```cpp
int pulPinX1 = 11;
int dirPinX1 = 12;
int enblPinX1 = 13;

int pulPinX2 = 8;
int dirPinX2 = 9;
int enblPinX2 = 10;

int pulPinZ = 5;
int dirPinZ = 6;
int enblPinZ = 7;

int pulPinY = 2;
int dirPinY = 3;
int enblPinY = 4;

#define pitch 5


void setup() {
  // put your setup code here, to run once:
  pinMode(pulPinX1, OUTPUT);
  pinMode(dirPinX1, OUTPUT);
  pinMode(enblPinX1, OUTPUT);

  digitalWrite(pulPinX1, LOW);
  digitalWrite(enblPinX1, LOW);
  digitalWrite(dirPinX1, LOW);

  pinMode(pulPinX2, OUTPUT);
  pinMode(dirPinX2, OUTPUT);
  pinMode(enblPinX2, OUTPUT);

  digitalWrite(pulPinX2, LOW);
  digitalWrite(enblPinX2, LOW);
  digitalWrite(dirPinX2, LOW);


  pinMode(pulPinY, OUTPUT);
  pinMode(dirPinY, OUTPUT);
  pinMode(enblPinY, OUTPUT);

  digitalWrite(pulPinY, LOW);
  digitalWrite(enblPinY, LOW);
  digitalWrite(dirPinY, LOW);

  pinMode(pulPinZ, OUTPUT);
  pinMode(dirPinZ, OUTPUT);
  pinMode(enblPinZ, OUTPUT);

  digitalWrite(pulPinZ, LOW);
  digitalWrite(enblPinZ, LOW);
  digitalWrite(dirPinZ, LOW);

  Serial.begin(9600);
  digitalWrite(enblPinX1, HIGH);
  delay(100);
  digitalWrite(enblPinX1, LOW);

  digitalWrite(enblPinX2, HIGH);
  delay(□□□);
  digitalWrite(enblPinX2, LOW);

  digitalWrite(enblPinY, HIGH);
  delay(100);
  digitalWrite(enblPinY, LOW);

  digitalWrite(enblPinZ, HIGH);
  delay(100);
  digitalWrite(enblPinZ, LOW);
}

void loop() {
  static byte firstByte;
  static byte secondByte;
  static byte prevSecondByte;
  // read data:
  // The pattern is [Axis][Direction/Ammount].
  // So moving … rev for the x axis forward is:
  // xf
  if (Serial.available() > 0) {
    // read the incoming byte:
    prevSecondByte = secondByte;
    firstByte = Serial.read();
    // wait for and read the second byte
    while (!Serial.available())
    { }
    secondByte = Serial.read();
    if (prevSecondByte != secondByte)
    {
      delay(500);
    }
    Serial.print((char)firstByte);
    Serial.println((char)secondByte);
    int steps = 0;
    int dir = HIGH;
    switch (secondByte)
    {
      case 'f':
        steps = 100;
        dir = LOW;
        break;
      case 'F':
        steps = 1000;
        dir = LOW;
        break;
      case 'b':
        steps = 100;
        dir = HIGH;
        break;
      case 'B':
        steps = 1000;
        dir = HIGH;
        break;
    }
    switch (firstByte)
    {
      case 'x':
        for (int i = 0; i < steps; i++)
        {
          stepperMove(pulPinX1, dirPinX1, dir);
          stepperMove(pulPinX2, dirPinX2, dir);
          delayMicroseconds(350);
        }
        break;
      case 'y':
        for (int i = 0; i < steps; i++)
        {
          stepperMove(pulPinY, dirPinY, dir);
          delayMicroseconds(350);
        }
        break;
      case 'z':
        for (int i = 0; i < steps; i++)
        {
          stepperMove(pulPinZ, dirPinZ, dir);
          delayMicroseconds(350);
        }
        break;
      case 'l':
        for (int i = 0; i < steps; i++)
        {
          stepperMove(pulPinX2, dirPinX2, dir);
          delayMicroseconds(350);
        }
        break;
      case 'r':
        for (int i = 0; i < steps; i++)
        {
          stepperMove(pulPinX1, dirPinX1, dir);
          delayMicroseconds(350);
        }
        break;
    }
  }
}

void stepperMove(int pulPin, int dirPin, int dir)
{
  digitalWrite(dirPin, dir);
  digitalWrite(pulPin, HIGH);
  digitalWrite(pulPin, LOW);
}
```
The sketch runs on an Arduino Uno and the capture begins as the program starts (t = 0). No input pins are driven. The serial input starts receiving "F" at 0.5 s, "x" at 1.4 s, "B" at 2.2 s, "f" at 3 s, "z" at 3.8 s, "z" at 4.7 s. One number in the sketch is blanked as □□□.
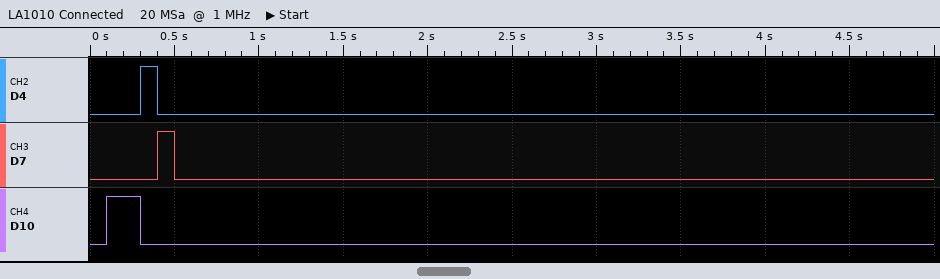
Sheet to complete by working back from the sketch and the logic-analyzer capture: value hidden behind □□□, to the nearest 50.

200
